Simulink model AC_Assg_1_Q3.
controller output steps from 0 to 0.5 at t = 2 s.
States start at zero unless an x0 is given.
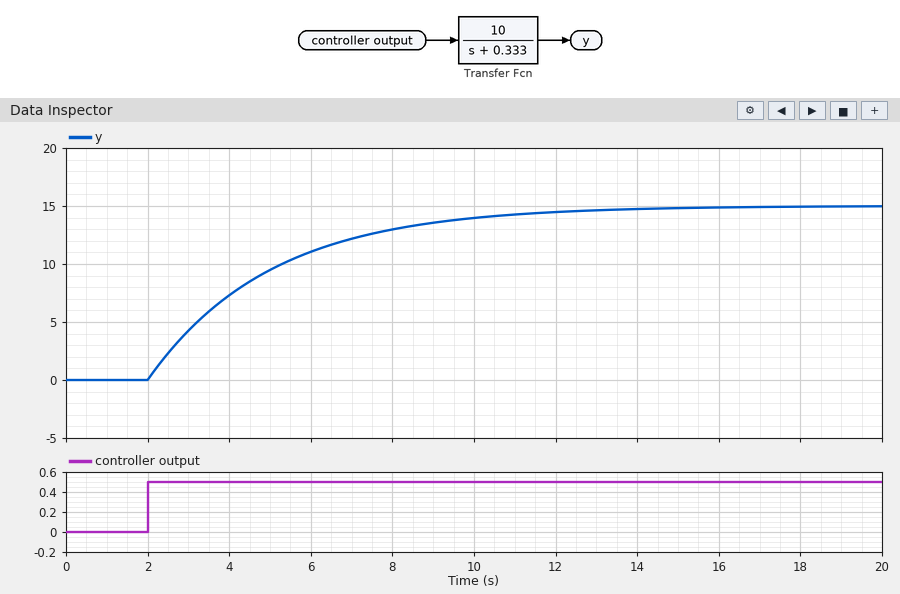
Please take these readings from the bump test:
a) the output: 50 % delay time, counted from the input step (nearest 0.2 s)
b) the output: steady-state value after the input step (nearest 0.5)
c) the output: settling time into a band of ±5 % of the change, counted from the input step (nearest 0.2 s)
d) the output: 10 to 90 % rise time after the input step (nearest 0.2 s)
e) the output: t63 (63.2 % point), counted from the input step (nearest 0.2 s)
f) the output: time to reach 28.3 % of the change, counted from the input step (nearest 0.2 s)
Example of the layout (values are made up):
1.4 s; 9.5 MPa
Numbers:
2.0 s; 15.0; 9.0 s; 6.6 s; 3.0 s; 1.0 s
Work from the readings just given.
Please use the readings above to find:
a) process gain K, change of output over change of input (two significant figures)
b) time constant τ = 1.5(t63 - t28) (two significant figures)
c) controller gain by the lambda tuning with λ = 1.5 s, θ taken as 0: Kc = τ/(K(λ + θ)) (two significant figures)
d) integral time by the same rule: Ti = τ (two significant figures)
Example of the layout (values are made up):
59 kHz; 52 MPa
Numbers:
30; 3.0 s; 0.067; 3.0 s
